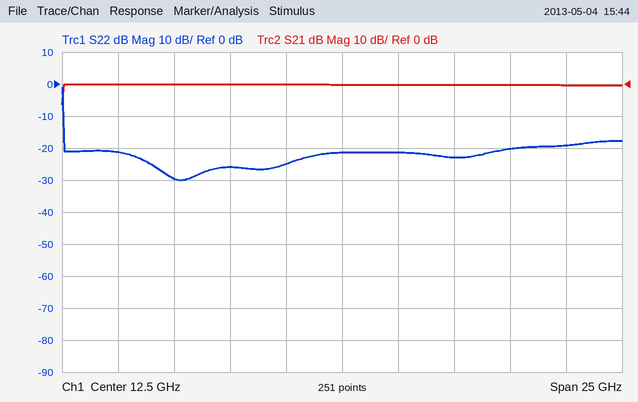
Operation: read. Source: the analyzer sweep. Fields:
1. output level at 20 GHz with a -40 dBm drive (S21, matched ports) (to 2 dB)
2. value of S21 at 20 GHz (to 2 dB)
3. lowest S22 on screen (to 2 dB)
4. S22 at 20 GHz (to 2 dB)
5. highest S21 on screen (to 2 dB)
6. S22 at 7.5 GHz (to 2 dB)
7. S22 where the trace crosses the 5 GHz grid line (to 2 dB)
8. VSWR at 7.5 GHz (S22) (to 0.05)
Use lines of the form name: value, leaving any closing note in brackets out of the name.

output level at 20 GHz with a -40 dBm drive (S21, matched ports): -40 dBm
value of S21 at 20 GHz: 0 dB
lowest S22 on screen: -30 dB
S22 at 20 GHz: -20 dB
highest S21 on screen: 0 dB
S22 at 7.5 GHz: -26 dB
S22 where the trace crosses the 5 GHz grid line: -30 dB
VSWR at 7.5 GHz (S22): 1.10
